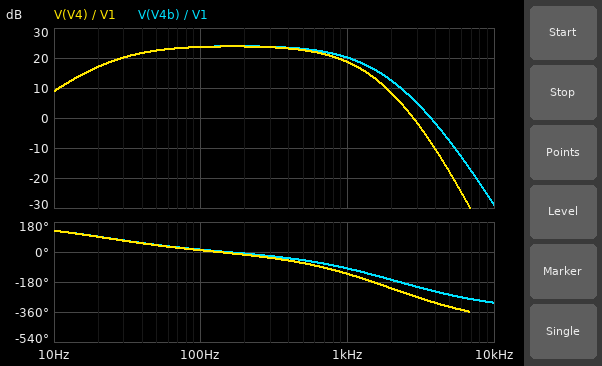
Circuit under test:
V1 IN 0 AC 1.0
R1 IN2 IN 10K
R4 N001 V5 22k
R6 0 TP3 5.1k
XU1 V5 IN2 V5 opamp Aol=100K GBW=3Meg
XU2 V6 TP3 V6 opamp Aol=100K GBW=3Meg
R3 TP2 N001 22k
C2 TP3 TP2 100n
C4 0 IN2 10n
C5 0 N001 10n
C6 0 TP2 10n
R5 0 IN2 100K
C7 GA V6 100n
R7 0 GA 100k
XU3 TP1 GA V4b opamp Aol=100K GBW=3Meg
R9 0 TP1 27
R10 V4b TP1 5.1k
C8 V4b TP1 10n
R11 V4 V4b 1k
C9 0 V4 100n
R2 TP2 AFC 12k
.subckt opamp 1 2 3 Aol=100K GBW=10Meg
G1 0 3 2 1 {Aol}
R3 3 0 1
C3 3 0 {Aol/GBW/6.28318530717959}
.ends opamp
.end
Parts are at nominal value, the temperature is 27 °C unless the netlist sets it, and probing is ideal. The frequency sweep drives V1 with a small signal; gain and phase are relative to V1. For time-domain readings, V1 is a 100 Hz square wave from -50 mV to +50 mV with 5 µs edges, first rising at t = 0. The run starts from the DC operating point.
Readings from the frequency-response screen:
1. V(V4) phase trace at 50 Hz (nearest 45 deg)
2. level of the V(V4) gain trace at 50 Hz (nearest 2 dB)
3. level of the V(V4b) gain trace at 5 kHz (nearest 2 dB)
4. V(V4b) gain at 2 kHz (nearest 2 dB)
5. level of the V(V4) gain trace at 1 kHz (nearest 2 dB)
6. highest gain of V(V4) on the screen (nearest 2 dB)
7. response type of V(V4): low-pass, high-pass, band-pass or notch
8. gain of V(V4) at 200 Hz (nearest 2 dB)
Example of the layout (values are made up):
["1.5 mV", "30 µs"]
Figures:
["45 deg", "22 dB", "-8 dB", "12 dB", "18 dB", "24 dB", "band-pass", "24 dB"]
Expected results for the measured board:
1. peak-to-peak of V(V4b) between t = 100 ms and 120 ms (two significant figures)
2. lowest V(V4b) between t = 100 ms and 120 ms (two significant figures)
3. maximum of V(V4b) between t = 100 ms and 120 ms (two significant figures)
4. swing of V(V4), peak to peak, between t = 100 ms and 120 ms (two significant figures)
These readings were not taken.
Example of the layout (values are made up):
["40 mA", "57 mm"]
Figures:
["2.3 V", "-1.2 V", "1.2 V", "2.3 V"]
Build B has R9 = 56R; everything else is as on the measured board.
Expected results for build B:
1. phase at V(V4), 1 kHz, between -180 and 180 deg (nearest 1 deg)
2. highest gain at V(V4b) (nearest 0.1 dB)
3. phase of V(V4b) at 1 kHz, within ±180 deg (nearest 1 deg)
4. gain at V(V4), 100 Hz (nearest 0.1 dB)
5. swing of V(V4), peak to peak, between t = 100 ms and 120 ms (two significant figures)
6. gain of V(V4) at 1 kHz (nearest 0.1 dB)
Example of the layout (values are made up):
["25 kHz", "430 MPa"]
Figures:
["-129 deg", "17.6 dB", "-97 deg", "17.4 dB", "1.1 V", "12.5 dB"]
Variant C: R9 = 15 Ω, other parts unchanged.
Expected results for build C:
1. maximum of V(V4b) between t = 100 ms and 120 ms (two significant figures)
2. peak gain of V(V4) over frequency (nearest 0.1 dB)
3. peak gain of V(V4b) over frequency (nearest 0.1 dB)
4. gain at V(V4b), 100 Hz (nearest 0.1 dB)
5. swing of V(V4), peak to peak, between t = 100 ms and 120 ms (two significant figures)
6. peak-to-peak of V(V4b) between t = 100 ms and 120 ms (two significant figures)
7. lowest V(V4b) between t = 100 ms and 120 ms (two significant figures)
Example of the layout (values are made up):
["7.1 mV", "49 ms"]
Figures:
["2.1 V", "28.9 dB", "29.0 dB", "28.8 dB", "4.1 V", "4.2 V", "-2.1 V"]
